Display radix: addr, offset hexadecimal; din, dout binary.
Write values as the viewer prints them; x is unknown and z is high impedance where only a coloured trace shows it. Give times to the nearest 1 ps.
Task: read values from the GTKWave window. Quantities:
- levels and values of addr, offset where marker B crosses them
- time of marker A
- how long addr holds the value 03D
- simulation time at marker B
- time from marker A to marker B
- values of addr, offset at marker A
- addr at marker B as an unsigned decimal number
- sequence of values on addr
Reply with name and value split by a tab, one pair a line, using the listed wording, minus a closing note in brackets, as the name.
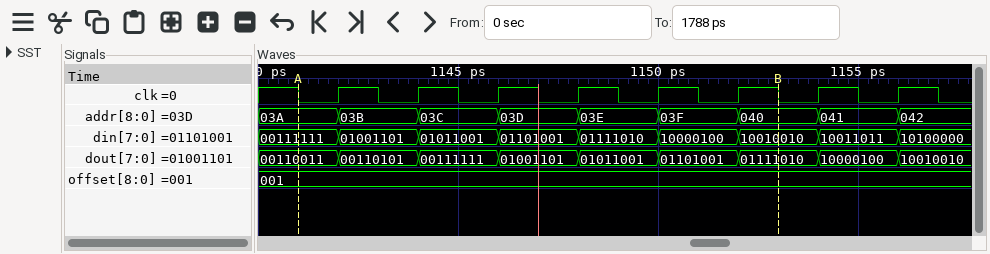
levels and values of addr, offset where marker B crosses them	addr=040, offset=001
time of marker A	1141 ps
how long addr holds the value 03D	2 ps
simulation time at marker B	1153 ps
time from marker A to marker B	12 ps
values of addr, offset at marker A	addr=03A, offset=001
addr at marker B as an unsigned decimal number	64
sequence of values on addr	03A, 03B, 03C, 03D, 03E, 03F, 040, 041, 042
